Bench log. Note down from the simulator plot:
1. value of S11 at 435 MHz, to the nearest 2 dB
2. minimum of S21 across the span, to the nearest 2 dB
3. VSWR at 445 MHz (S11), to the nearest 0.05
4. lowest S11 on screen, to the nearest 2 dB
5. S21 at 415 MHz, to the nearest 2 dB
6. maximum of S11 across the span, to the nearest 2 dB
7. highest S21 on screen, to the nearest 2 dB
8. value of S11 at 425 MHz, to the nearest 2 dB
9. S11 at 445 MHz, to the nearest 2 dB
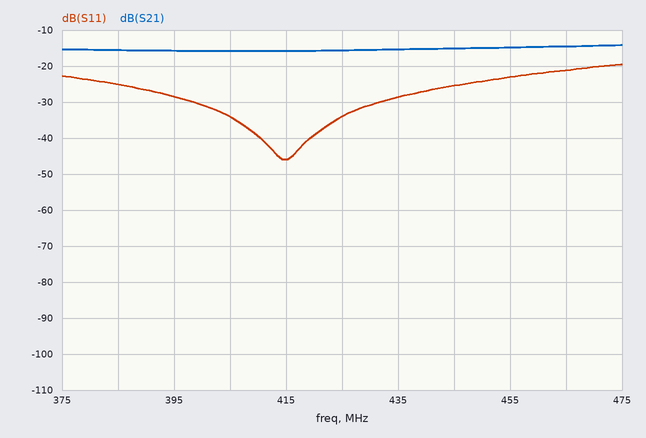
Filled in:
-28 dB
-16 dB
1.10
-46 dB
-16 dB
-20 dB
-14 dB
-34 dB
-26 dB
